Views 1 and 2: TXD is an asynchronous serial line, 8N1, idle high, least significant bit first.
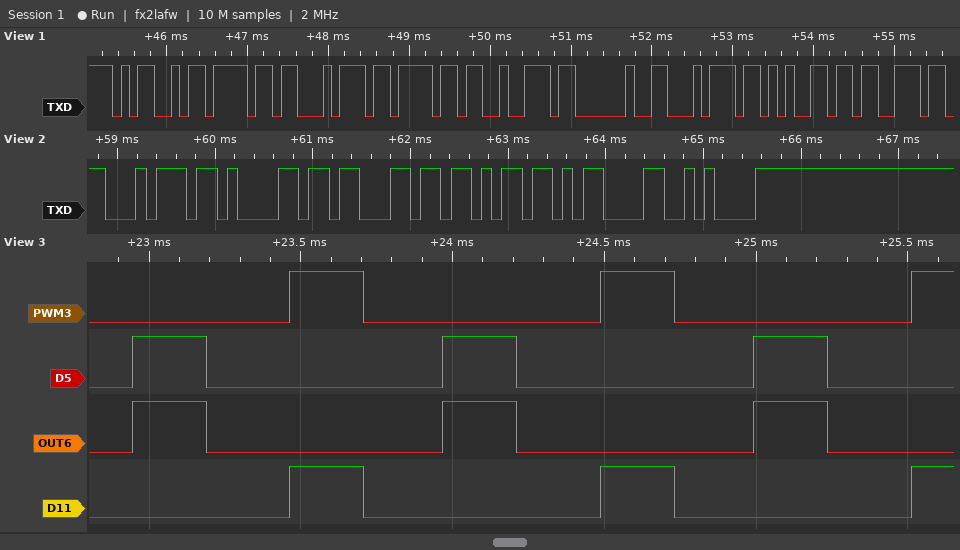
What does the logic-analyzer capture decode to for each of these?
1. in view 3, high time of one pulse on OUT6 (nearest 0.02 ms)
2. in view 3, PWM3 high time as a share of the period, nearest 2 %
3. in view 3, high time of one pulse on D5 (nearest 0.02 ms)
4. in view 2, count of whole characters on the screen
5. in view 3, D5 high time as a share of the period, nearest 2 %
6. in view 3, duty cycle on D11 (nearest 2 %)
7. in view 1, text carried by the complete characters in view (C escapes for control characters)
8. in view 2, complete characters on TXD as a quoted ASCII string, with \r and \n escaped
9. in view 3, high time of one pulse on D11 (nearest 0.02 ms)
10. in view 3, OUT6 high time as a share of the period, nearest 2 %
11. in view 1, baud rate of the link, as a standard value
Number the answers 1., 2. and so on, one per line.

1. 0.24 ms
2. 24 %
3. 0.24 ms
4. 6
5. 24 %
6. 24 %
7. "Motor tes"
8. "tack\r\n"
9. 0.24 ms
10. 24 %
11. 9600 baud
